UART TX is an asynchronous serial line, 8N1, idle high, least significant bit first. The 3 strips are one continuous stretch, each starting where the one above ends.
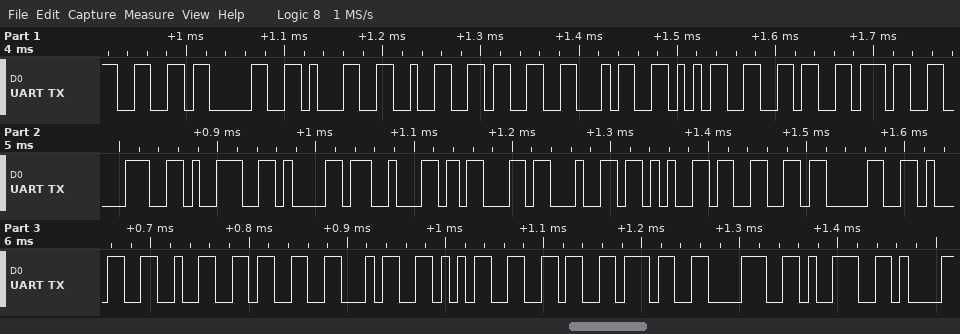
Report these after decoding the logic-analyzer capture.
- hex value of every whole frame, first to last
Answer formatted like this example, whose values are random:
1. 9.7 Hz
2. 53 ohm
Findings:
1. 0x66 0x30 0x31 0x32 0x33 0x34 0x35 0x36 0x37 0x38 0x39 0x61 0x62 0x63 0x64 0x65 0x66 0x30 0x31 0x32 0x33 0x34 0x35 0x36 0x37 0x38 0x39
